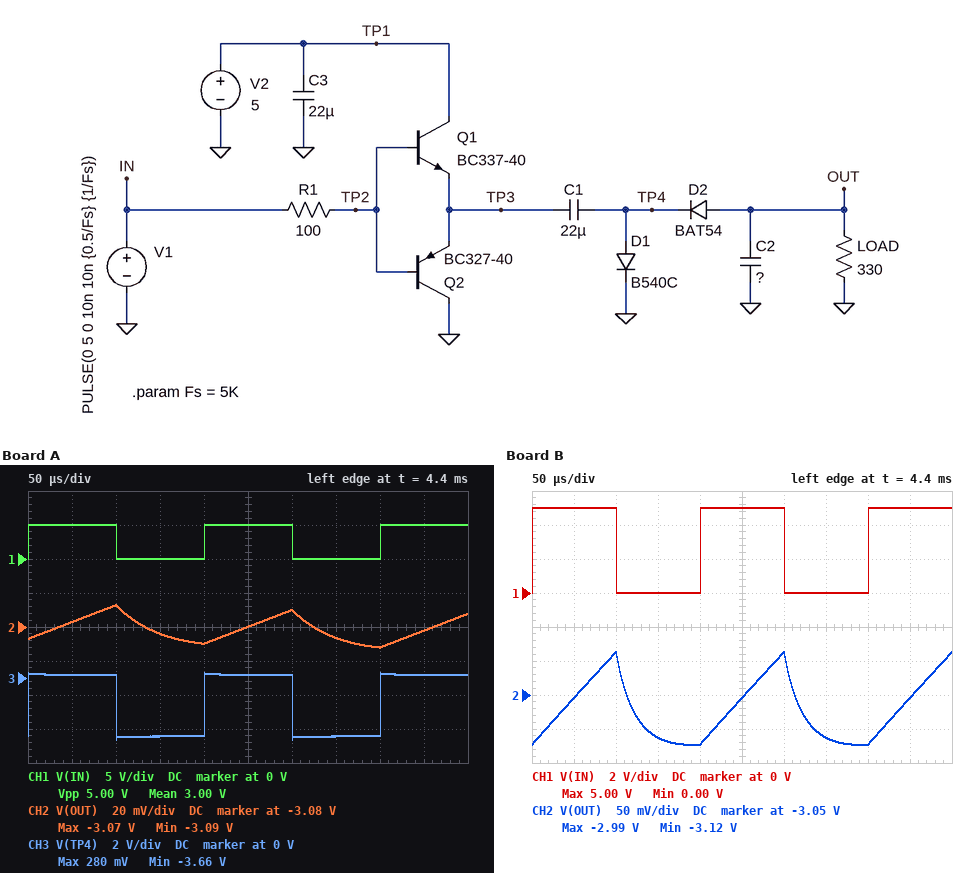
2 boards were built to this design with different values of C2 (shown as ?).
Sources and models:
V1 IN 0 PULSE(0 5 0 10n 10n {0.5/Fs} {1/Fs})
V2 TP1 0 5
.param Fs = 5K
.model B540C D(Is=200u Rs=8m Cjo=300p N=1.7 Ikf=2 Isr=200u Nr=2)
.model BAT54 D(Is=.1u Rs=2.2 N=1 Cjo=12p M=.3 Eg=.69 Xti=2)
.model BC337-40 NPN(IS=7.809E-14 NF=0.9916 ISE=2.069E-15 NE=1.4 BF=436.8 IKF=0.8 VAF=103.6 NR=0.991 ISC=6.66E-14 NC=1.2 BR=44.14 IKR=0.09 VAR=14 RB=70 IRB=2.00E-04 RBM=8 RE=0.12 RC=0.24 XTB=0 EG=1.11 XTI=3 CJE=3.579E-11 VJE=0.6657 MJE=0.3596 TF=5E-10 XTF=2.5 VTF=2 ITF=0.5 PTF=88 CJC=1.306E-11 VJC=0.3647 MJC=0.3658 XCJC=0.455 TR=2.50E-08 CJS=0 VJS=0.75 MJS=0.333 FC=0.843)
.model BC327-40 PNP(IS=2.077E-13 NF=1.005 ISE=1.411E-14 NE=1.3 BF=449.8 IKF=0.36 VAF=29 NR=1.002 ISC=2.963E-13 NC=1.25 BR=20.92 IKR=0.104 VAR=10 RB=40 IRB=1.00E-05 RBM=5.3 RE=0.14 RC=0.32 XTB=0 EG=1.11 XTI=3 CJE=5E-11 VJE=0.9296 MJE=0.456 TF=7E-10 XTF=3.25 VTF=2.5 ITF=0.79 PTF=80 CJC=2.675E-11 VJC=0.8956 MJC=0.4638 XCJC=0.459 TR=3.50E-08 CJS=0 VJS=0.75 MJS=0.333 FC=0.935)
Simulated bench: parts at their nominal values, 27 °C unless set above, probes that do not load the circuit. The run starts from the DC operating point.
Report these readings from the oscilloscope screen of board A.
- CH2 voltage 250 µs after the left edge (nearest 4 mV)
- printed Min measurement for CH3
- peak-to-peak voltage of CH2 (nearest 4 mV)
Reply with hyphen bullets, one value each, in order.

- -3.080 V
- -3.66 V
- 24 mV
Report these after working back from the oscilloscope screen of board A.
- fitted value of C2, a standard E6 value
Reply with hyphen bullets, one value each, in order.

- 47 µF
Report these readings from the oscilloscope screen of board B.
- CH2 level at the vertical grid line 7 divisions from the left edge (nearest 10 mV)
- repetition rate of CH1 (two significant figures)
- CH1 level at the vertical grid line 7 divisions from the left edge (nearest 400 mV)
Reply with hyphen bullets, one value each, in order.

- -3.11 V
- 5.0 kHz
- 0 V
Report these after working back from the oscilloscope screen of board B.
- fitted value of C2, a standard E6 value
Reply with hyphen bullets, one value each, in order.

- 6.8 µF
